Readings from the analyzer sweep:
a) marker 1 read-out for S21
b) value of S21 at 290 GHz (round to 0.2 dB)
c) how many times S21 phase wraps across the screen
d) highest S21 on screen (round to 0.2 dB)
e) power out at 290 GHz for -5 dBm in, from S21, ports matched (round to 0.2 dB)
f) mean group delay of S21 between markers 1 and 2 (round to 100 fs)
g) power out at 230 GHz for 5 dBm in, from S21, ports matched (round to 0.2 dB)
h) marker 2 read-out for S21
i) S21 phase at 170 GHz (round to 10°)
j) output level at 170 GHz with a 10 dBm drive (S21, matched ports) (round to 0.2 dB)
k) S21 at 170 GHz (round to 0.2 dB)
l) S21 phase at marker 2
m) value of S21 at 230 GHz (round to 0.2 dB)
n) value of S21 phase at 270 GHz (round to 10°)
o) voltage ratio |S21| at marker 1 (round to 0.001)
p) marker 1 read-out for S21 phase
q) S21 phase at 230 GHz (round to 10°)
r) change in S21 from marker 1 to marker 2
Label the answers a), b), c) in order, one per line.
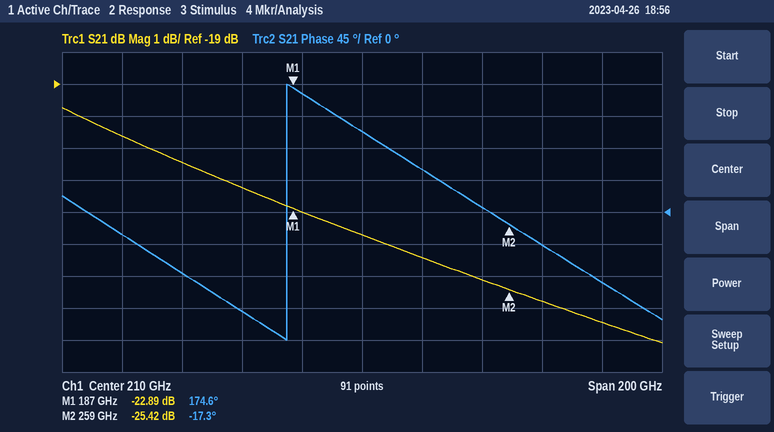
a) -22.89 dB
b) -26.4 dB
c) 1
d) -19.8 dB
e) -31.4 dBm
f) 7.4 ps
g) -19.4 dBm
h) -25.42 dB
i) -140°
j) -12.2 dBm
k) -22.2 dB
l) -17.3°
m) -24.4 dB
n) -50°
o) 0.072
p) 174.6°
q) 60°
r) -2.53 dB
